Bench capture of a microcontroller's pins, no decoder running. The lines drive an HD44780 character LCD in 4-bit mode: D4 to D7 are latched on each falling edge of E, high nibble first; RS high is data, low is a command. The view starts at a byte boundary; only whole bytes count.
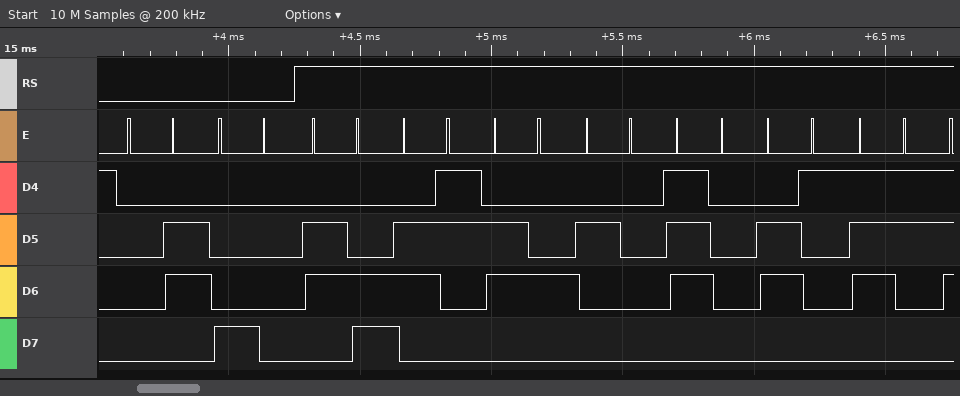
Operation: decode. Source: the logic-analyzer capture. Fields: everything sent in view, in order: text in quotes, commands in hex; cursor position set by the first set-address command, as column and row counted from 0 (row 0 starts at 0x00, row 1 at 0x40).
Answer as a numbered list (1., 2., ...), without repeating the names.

1. 0x06 0x80 "lcd pas"
2. column 0, row 0
